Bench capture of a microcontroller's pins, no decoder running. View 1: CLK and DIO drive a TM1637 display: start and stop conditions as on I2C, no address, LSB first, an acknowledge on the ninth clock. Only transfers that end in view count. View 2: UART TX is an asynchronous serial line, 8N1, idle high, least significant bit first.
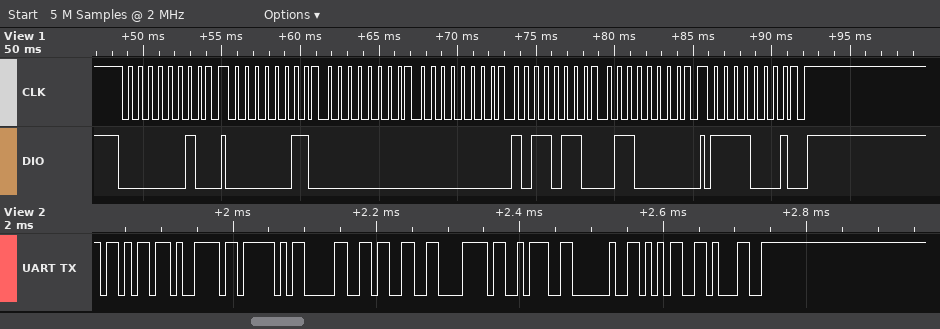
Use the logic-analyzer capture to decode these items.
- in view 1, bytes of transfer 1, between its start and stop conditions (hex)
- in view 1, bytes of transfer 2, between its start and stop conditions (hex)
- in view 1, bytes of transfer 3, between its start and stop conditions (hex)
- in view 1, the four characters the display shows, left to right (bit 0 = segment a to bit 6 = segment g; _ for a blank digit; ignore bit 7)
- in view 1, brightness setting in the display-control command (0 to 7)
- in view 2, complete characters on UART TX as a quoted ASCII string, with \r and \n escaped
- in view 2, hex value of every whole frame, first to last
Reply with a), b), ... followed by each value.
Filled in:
a) 40
b) C0 00 00 6D 06
c) 8F
d) __51
e) 7
f) "ky_03x: 51"
g) 6B 79 5F 30 33 78 3A 20 35 31
